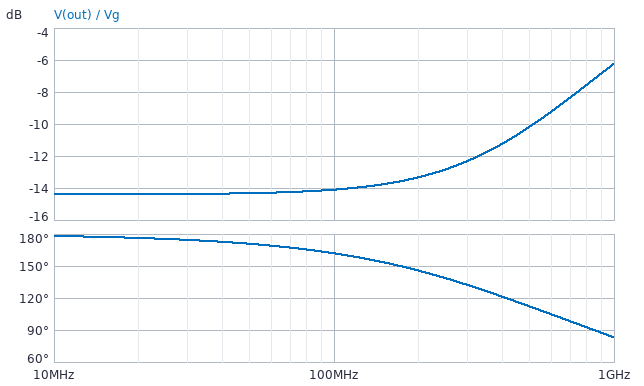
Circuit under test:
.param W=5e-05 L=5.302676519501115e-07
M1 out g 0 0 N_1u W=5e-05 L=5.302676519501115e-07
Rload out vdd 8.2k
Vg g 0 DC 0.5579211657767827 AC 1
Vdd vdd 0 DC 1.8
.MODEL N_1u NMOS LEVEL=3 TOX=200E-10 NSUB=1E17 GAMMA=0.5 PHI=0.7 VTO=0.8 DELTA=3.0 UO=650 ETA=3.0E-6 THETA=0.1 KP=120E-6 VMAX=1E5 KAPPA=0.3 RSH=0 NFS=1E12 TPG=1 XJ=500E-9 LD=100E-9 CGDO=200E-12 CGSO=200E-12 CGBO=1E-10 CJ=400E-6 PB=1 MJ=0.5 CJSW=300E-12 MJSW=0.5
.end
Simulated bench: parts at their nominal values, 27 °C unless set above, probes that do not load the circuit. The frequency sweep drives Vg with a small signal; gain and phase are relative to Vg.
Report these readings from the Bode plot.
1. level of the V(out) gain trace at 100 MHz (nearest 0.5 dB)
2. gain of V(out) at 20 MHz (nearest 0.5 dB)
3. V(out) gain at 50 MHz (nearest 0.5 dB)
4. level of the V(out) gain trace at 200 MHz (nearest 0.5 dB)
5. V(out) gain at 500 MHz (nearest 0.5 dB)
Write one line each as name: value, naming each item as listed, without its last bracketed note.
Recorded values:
level of the V(out) gain trace at 100 MHz: -14.0 dB
gain of V(out) at 20 MHz: -14.5 dB
V(out) gain at 50 MHz: -14.5 dB
level of the V(out) gain trace at 200 MHz: -13.5 dB
V(out) gain at 500 MHz: -10.0 dB
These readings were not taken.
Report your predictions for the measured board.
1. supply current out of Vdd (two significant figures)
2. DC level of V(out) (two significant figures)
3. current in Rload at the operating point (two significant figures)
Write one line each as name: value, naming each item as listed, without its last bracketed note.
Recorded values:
supply current out of Vdd: 1.3 µA
DC level of V(out): 1.8 V
current in Rload at the operating point: 1.3 µA
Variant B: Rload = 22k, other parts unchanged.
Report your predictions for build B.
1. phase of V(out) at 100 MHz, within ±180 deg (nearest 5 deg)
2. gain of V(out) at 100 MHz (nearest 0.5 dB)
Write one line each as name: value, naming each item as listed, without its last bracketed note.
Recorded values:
phase of V(out) at 100 MHz, within ±180 deg: 155 deg
gain of V(out) at 100 MHz: -5.5 dB
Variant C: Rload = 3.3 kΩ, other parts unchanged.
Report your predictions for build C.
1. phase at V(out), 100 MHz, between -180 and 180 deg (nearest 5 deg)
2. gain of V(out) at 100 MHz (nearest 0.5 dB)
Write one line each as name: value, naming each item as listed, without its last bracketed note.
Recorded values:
phase at V(out), 100 MHz, between -180 and 180 deg: 165 deg
gain of V(out) at 100 MHz: -22.0 dB
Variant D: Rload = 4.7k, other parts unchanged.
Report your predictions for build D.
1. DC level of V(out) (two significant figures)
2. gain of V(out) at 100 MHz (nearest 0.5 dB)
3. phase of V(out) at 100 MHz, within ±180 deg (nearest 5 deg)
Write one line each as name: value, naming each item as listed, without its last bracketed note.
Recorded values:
DC level of V(out): 1.8 V
gain of V(out) at 100 MHz: -19.0 dB
phase of V(out) at 100 MHz, within ±180 deg: 165 deg
